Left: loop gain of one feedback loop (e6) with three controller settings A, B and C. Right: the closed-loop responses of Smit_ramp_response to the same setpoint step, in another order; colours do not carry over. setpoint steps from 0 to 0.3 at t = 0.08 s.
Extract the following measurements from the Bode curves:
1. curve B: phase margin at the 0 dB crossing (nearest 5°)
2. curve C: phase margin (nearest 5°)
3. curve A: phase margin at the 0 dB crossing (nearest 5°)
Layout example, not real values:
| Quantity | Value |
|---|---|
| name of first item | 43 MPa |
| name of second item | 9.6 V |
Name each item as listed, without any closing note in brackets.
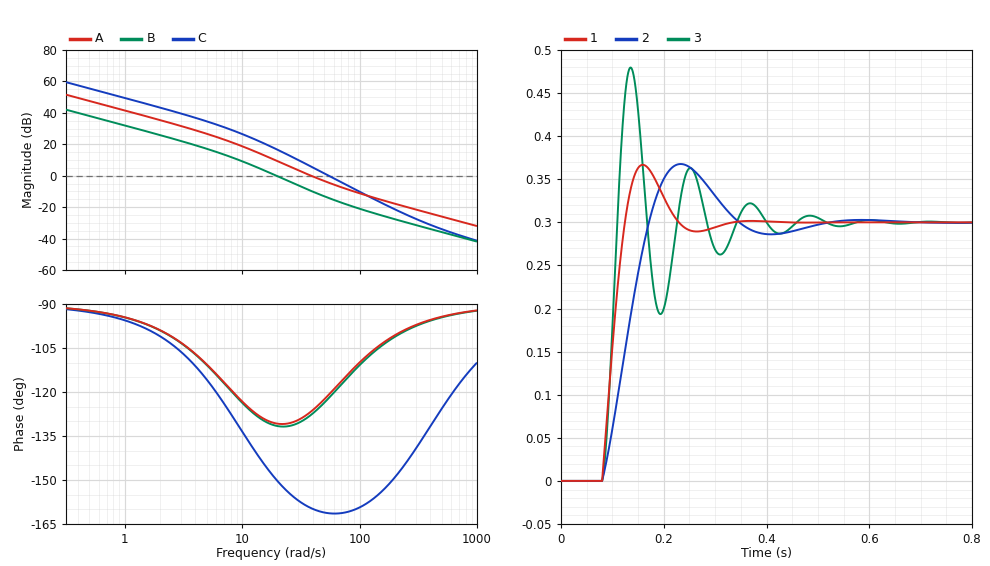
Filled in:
| Quantity | Value |
|---|---|
| curve B: phase margin at the 0 dB crossing | 50° |
| curve C: phase margin | 20° |
| curve A: phase margin at the 0 dB crossing | 55° |
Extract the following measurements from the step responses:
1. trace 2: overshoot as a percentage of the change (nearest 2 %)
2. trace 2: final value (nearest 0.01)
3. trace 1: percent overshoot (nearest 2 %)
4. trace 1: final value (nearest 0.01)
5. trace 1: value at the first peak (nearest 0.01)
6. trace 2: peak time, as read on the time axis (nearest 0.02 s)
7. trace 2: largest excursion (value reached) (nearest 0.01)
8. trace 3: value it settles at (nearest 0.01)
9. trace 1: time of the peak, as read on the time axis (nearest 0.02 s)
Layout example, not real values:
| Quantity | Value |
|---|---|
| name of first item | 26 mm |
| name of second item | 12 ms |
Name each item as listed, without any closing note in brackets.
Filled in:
| Quantity | Value |
|---|---|
| trace 2: overshoot as a percentage of the change | 22 % |
| trace 2: final value | 0.30 |
| trace 1: percent overshoot | 22 % |
| trace 1: final value | 0.30 |
| trace 1: value at the first peak | 0.37 |
| trace 2: peak time, as read on the time axis | 0.24 s |
| trace 2: largest excursion (value reached) | 0.37 |
| trace 3: value it settles at | 0.30 |
| trace 1: time of the peak, as read on the time axis | 0.16 s |
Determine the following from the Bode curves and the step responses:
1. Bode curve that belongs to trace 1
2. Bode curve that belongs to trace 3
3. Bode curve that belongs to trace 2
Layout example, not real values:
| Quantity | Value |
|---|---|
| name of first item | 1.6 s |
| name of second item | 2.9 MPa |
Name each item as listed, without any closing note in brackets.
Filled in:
| Quantity | Value |
|---|---|
| Bode curve that belongs to trace 1 | A |
| Bode curve that belongs to trace 3 | C |
| Bode curve that belongs to trace 2 | B |
